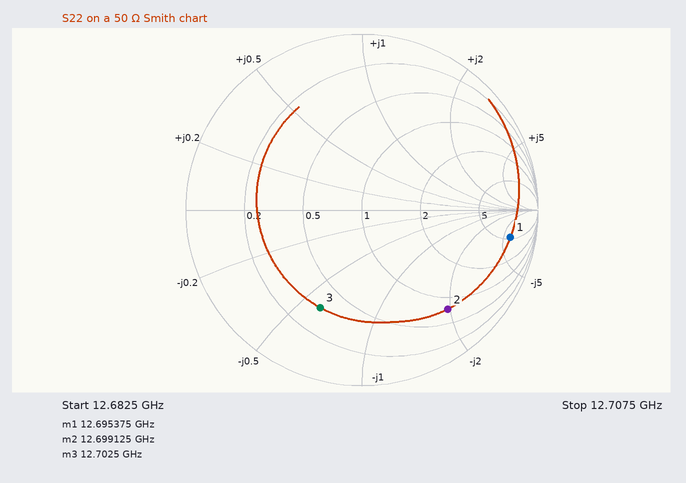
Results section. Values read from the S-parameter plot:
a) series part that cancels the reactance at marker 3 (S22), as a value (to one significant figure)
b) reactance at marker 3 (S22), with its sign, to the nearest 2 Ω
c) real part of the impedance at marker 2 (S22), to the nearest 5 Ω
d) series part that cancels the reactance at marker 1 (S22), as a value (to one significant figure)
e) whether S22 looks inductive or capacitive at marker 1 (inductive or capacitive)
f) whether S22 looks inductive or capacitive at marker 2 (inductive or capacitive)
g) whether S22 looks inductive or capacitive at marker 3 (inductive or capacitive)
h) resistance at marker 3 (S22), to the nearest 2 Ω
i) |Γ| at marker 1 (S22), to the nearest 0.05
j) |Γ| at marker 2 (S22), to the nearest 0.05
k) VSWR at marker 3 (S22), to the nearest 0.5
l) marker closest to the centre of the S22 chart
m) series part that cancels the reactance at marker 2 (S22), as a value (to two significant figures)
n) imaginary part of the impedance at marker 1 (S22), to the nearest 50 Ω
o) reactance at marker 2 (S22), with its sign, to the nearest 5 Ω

400 pH
-30 Ω
40 Ω
4 nH
capacitive
capacitive
capacitive
18 Ω
0.85
0.75
4.0
marker 3
1.2 nH
-300 Ω
-95 Ω
